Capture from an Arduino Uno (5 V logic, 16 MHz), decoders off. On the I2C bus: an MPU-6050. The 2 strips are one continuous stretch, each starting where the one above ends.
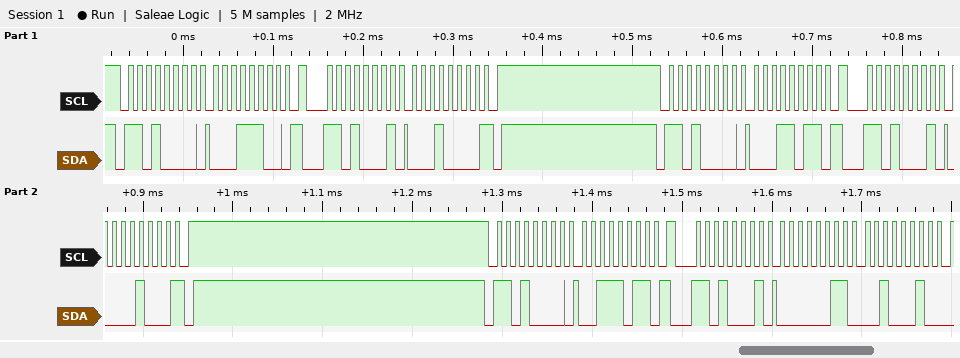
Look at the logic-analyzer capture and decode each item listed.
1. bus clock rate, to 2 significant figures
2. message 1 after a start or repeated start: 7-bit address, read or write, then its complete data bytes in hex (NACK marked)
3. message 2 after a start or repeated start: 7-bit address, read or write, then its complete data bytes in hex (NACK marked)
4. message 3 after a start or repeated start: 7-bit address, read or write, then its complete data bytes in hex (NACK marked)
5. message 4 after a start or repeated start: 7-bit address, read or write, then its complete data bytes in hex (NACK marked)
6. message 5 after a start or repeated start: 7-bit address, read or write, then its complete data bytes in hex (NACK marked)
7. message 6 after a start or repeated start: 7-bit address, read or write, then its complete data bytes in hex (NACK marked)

100 kHz
0x68 write: 1C
0x68 read: 10 NACK
0x68 write: 1B
0x68 read: 08 NACK
0x68 write: 3B
0x68 read: 03 22
